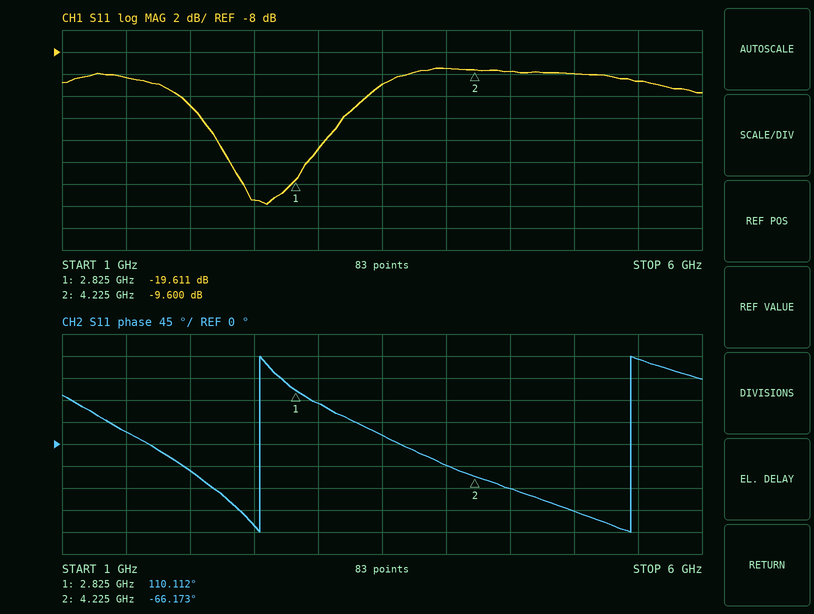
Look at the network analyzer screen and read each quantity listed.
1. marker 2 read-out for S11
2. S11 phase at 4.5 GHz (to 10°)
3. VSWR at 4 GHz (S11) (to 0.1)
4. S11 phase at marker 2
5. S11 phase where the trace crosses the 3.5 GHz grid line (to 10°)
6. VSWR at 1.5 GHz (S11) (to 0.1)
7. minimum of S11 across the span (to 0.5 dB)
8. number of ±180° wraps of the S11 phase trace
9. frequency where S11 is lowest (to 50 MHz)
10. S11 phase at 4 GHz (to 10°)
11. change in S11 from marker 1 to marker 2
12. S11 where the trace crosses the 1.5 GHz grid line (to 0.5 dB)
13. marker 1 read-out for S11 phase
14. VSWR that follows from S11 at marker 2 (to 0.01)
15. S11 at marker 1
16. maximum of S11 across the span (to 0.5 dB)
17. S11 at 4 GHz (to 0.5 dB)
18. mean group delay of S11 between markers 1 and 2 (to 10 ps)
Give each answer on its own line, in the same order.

-9.600 dB
-90°
2.0
-66.173°
20°
1.9
-22.0 dB
2
2.60 GHz
-40°
10.011 dB
-10.5 dB
110.112°
1.99
-19.611 dB
-9.5 dB
-9.5 dB
350 ps
